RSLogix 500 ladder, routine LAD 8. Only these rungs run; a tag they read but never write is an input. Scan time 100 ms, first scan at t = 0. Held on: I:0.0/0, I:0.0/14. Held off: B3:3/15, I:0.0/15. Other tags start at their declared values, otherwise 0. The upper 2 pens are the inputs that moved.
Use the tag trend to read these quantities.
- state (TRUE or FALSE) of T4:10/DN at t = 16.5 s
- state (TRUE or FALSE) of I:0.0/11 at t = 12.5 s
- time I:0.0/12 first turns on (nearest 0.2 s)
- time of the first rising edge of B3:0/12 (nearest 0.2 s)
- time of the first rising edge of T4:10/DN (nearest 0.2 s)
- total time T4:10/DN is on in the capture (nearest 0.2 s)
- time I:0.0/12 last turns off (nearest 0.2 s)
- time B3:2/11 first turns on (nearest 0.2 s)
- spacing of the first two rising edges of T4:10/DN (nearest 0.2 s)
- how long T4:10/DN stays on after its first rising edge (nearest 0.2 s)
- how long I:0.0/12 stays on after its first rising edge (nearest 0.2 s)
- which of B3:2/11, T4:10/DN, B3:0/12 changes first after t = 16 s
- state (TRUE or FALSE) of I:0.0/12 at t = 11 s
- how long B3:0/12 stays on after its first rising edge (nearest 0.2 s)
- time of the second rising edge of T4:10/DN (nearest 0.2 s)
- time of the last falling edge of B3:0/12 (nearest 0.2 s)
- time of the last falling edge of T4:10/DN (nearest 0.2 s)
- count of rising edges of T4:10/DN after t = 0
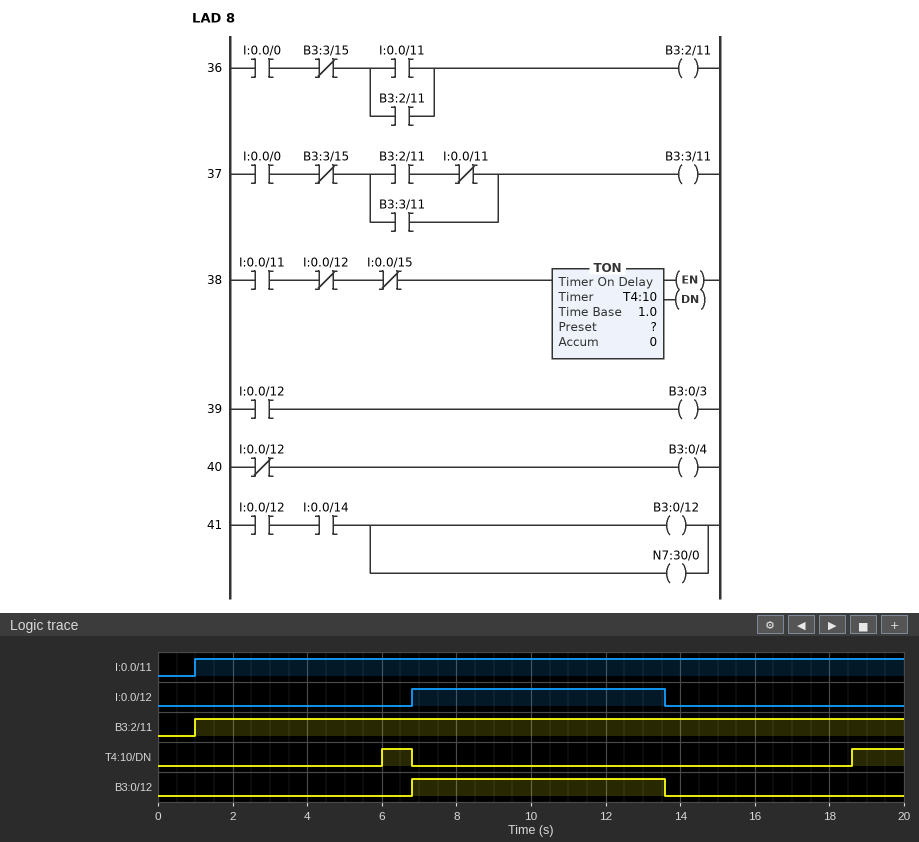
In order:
FALSE
TRUE
6.8 s
6.8 s
6.0 s
2.2 s
13.6 s
1.0 s
12.6 s
0.8 s
6.8 s
T4:10/DN
TRUE
6.8 s
18.6 s
13.6 s
6.8 s
2
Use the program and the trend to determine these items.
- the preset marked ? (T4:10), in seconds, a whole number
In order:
5 s
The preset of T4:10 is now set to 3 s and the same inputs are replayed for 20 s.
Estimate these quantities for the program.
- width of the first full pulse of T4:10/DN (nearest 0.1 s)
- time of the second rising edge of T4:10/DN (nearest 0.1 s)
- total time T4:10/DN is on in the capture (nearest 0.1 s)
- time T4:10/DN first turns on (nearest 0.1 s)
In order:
2.8 s
16.6 s
6.2 s
4.0 s
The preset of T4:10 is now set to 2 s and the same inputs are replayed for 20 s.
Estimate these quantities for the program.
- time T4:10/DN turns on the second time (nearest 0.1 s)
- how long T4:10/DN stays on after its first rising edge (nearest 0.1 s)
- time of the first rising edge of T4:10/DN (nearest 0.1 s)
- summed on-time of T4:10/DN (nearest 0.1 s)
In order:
15.6 s
3.8 s
3.0 s
8.2 s
